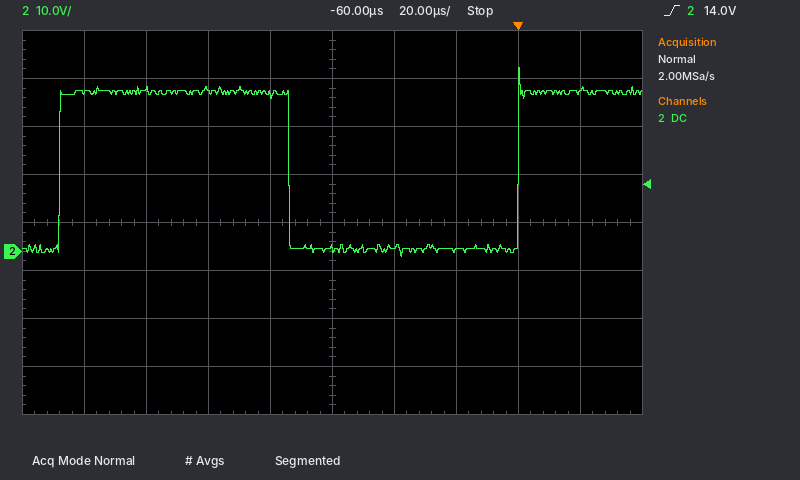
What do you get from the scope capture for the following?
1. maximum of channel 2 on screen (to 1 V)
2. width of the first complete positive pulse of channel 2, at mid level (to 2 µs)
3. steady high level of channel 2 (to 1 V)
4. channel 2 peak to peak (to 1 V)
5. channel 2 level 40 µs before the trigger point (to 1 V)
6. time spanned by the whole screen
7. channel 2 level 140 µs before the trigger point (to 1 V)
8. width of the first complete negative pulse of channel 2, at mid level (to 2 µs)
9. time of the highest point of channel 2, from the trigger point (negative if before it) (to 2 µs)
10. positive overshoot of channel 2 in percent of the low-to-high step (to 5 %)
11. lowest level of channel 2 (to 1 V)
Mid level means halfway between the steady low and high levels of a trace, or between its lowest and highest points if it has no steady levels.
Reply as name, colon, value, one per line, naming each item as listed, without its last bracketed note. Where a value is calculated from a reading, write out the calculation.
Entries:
maximum of channel 2 on screen: 38 V
width of the first complete positive pulse of channel 2, at mid level: 74 µs
steady high level of channel 2: 33 V
channel 2 peak to peak: 38 V − (-1 V) = 39 V
channel 2 level 40 µs before the trigger point: 1 V
time spanned by the whole screen: 200 µs
channel 2 level 140 µs before the trigger point: 33 V
width of the first complete negative pulse of channel 2, at mid level: 74 µs
time of the highest point of channel 2, from the trigger point (negative if before it): 0 µs
positive overshoot of channel 2 in percent of the low-to-high step: 15 %
lowest level of channel 2: -1 V
